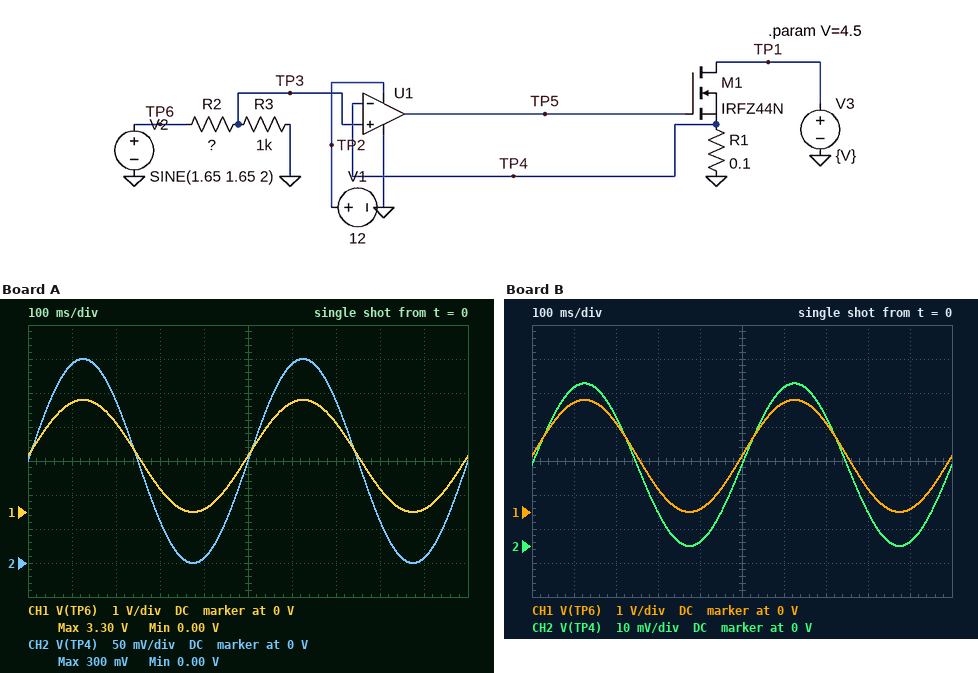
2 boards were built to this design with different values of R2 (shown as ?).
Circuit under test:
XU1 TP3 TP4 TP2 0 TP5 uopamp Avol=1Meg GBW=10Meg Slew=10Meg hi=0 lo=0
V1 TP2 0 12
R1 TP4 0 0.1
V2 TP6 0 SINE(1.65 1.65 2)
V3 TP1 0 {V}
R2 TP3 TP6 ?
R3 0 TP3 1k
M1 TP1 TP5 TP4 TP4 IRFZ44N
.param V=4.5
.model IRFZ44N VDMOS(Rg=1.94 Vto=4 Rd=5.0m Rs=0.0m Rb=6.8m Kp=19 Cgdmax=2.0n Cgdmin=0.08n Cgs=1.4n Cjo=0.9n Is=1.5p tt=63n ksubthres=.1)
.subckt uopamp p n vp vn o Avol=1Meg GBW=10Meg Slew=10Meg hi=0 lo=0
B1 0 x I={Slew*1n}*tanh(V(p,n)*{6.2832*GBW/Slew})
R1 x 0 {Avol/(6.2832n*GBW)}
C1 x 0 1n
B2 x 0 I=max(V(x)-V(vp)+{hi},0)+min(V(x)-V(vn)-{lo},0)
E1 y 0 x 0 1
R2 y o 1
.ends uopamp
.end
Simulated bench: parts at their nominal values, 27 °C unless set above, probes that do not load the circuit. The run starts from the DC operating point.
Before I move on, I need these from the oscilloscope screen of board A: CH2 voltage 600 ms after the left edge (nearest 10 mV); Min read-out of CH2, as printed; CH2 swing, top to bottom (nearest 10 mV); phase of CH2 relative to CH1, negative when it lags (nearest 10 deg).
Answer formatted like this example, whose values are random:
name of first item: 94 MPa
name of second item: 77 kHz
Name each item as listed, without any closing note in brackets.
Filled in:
CH2 voltage 600 ms after the left edge: 290 mV
Min read-out of CH2, as printed: 0.00 V
CH2 swing, top to bottom: 300 mV
phase of CH2 relative to CH1, negative when it lags: 0 deg
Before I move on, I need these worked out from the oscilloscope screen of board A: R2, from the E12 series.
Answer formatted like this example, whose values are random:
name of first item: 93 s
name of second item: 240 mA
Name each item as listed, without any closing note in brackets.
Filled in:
R2, from the E12 series: 10 kΩ
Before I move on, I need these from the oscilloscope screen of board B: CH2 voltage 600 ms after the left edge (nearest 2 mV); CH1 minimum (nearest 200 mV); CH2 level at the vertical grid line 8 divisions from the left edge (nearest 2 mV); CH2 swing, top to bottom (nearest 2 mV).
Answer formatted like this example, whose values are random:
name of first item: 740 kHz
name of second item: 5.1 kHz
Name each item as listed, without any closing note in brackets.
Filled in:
CH2 voltage 600 ms after the left edge: 46 mV
CH1 minimum: 0 V
CH2 level at the vertical grid line 8 divisions from the left edge: 10 mV
CH2 swing, top to bottom: 48 mV
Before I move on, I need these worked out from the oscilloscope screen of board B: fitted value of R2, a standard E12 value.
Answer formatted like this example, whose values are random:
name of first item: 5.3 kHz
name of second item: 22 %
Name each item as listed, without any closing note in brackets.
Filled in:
fitted value of R2, a standard E12 value: 68 kΩ
